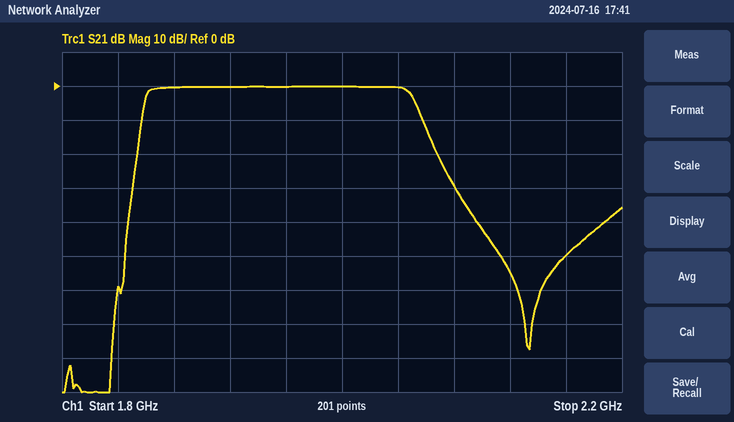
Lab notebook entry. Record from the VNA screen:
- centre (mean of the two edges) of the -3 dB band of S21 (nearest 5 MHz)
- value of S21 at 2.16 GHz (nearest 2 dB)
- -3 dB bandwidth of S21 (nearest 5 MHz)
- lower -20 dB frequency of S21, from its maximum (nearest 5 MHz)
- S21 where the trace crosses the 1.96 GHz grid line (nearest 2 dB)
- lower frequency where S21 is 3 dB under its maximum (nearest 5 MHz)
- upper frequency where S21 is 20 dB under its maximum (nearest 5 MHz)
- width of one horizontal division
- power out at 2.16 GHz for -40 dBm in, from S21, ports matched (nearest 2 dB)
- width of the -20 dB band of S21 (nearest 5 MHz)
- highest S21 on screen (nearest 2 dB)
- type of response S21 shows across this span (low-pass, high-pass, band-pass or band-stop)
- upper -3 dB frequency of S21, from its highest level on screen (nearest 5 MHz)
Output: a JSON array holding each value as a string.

["1.955 GHz", "-50 dB", "190 MHz", "1.855 GHz", "0 dB", "1.860 GHz", "2.070 GHz", "40 MHz", "-90 dBm", "215 MHz", "0 dB", "band-pass", "2.050 GHz"]
